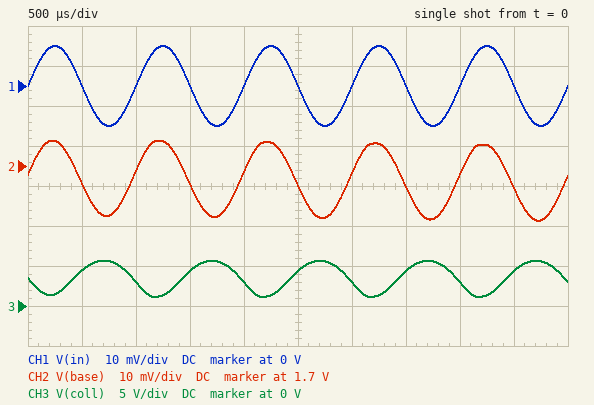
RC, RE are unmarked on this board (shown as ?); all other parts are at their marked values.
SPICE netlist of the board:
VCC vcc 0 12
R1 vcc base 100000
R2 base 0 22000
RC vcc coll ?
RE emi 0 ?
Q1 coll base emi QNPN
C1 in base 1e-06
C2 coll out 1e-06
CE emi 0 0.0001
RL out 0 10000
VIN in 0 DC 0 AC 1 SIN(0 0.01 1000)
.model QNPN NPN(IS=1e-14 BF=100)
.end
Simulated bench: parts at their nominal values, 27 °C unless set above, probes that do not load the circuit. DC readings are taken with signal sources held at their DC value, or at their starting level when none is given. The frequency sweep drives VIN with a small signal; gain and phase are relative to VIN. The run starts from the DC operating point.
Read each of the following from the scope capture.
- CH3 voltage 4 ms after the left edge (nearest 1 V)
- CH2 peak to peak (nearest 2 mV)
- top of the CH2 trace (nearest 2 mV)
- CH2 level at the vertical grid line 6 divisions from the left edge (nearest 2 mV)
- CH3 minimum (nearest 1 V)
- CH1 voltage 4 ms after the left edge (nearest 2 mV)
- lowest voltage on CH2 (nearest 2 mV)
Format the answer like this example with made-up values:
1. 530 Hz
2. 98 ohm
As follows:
1. 3 V
2. 20 mV
3. 1.706 V
4. 1.698 V
5. 1 V
6. 0 V
7. 1.686 V
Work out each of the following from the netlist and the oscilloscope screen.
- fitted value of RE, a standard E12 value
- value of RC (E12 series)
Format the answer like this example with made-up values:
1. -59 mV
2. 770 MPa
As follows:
1. 390 Ω
2. 3.3 kΩ
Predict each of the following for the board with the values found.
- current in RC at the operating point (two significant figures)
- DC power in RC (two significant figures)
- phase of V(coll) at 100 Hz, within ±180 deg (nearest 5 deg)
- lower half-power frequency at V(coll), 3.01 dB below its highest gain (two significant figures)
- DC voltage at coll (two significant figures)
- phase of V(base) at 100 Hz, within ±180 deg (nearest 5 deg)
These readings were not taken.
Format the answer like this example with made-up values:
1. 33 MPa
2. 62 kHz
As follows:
1. 2.6 mA
2. 22 mW
3. -110 deg
4. 330 Hz
5. 3.5 V
6. 20 deg
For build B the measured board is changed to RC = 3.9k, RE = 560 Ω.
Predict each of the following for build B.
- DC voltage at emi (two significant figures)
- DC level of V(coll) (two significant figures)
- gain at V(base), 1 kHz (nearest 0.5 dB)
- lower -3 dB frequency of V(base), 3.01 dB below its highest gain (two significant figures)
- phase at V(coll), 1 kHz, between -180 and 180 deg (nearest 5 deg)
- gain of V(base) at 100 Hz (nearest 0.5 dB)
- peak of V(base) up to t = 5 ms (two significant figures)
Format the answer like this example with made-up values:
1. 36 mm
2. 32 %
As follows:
1. 1.1 V
2. 4.2 V
3. 0 dB
4. 180 Hz
5. -165 deg
6. -4.5 dB
7. 1.8 V
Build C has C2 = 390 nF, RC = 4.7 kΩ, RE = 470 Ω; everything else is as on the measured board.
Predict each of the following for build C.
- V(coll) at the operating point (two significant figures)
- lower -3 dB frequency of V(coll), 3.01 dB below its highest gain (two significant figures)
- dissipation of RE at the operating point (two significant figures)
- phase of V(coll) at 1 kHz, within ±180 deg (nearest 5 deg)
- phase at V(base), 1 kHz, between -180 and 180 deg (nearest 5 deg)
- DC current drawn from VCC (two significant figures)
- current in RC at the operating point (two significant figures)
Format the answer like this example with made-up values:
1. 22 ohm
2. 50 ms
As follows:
1. 1.3 V
2. 440 Hz
3. 2.5 mW
4. -155 deg
5. 15 deg
6. 2.4 mA
7. 2.3 mA
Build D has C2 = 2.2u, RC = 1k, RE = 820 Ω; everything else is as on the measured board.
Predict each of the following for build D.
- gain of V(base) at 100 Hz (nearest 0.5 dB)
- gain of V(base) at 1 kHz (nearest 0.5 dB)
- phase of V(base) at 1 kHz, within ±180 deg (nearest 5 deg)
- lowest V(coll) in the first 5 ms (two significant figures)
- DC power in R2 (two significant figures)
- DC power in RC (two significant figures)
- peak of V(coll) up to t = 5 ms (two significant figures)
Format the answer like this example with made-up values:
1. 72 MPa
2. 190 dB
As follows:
1. -4.0 dB
2. 0 dB
3. 5 deg
4. 10 V
5. 160 µW
6. 2.2 mW
7. 11 V
